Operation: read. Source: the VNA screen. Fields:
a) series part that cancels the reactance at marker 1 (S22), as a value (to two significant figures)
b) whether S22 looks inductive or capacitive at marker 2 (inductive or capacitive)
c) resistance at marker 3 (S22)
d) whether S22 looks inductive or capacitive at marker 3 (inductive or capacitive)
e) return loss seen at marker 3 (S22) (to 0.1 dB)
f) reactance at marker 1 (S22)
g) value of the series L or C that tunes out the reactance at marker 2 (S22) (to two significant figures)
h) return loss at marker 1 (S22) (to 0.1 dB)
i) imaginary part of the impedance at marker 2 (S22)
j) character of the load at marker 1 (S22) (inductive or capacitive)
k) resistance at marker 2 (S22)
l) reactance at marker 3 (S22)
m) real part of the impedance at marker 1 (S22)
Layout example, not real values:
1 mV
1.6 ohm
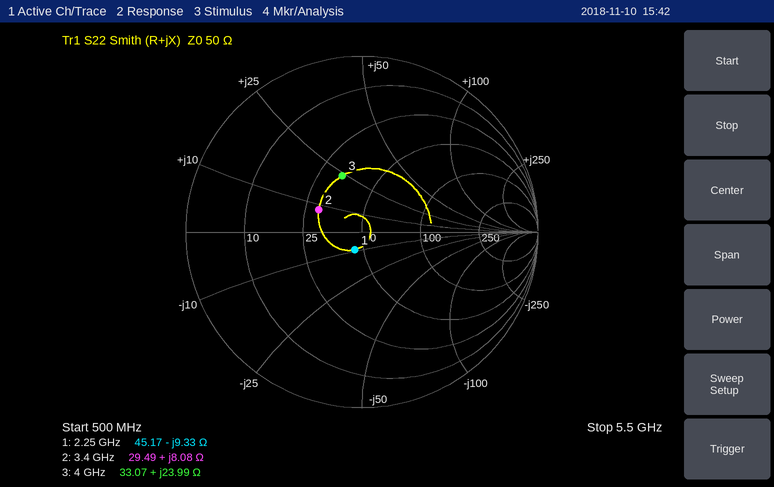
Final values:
660 pH
inductive
33.07 Ω
inductive
9.4 dB
-9.33 Ω
5.8 pF
19.2 dB
+8.08 Ω
capacitive
29.49 Ω
+23.99 Ω
45.17 Ω
